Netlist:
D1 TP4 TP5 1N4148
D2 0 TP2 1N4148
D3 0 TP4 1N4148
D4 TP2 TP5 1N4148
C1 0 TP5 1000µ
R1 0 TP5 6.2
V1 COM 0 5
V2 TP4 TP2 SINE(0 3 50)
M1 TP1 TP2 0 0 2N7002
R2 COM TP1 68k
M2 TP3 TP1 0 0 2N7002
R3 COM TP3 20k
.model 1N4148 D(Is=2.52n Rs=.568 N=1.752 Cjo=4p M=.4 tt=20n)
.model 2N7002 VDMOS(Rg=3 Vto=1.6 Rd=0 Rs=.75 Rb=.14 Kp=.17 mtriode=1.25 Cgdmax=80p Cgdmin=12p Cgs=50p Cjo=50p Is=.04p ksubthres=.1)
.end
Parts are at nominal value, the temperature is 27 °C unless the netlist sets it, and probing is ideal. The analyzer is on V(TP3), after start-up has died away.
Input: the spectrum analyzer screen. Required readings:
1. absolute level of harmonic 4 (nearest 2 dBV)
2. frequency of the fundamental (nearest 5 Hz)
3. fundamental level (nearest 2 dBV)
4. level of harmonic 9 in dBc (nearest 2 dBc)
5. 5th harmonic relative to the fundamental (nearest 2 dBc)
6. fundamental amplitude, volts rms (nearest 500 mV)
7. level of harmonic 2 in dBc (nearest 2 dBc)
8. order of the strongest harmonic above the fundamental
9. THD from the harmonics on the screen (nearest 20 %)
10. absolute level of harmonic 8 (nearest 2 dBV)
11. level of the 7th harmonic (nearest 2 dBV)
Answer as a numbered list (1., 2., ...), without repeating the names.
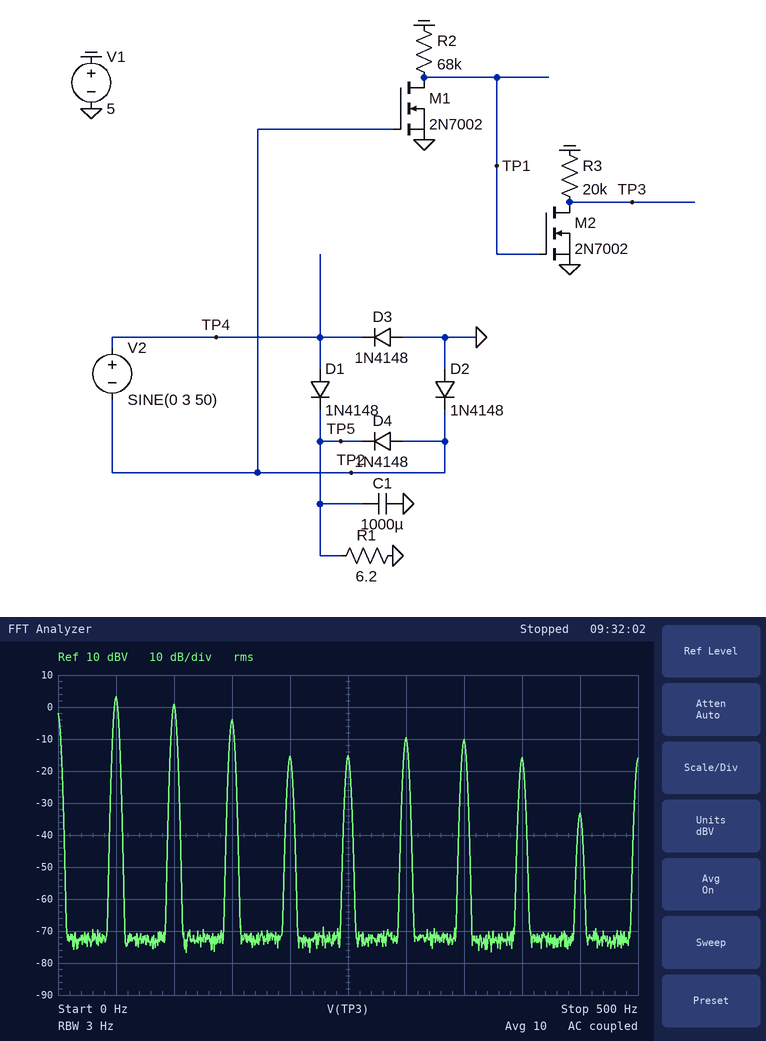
1. -16 dBV
2. 50 Hz
3. 4 dBV
4. -36 dBc
5. -18 dBc
6. 1.5 V
7. -2 dBc
8. 2
9. 100 %
10. -16 dBV
11. -10 dBV
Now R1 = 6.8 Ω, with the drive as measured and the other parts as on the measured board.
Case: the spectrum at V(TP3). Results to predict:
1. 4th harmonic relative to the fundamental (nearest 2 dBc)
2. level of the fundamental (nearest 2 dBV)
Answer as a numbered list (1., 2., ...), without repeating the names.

1. -20 dBc
2. 4 dBV
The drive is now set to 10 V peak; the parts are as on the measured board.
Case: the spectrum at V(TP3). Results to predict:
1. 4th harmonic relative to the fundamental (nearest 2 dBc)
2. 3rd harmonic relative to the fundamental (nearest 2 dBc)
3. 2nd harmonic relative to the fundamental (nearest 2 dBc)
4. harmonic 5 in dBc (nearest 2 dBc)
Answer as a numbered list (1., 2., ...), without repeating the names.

1. -32 dBc
2. -10 dBc
3. -32 dBc
4. -14 dBc
